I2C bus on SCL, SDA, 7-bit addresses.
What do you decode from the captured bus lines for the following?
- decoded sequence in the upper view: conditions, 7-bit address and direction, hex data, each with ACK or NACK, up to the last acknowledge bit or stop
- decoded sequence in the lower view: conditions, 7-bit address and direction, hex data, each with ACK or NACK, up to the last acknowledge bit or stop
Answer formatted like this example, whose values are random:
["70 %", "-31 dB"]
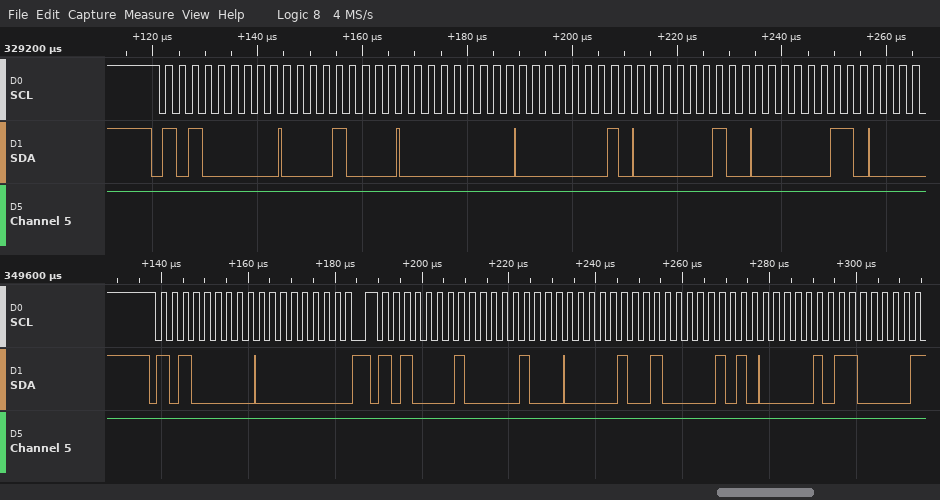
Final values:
["start, address 50 write ACK, 08 ACK, 00 ACK, 01 ACK, 02 ACK, 03 ACK", "start, address 50 write ACK, 00 ACK, repeated start, address 50 read ACK, 08 ACK, 09 ACK, 0A ACK, 0B ACK"]
